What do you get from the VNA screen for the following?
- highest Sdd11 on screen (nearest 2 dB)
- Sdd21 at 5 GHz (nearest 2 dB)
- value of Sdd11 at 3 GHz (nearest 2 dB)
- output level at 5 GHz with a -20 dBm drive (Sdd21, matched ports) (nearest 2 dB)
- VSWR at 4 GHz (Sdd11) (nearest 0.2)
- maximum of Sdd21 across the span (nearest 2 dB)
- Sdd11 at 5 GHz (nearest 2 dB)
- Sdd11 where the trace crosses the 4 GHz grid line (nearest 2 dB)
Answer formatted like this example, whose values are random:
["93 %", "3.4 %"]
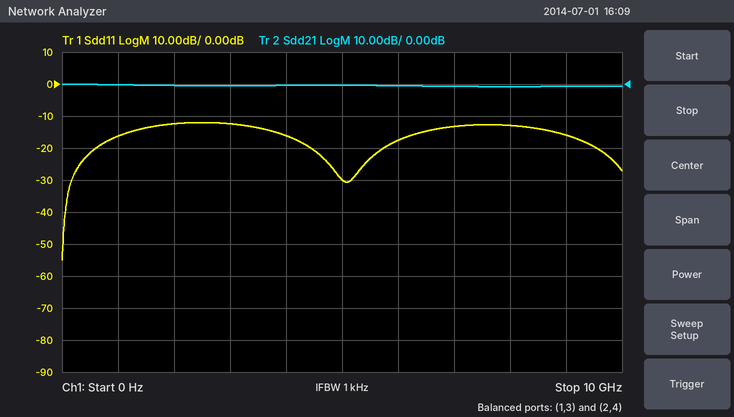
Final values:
["-12 dB", "0 dB", "-12 dB", "-20 dBm", "1.4", "0 dB", "-30 dB", "-16 dB"]
